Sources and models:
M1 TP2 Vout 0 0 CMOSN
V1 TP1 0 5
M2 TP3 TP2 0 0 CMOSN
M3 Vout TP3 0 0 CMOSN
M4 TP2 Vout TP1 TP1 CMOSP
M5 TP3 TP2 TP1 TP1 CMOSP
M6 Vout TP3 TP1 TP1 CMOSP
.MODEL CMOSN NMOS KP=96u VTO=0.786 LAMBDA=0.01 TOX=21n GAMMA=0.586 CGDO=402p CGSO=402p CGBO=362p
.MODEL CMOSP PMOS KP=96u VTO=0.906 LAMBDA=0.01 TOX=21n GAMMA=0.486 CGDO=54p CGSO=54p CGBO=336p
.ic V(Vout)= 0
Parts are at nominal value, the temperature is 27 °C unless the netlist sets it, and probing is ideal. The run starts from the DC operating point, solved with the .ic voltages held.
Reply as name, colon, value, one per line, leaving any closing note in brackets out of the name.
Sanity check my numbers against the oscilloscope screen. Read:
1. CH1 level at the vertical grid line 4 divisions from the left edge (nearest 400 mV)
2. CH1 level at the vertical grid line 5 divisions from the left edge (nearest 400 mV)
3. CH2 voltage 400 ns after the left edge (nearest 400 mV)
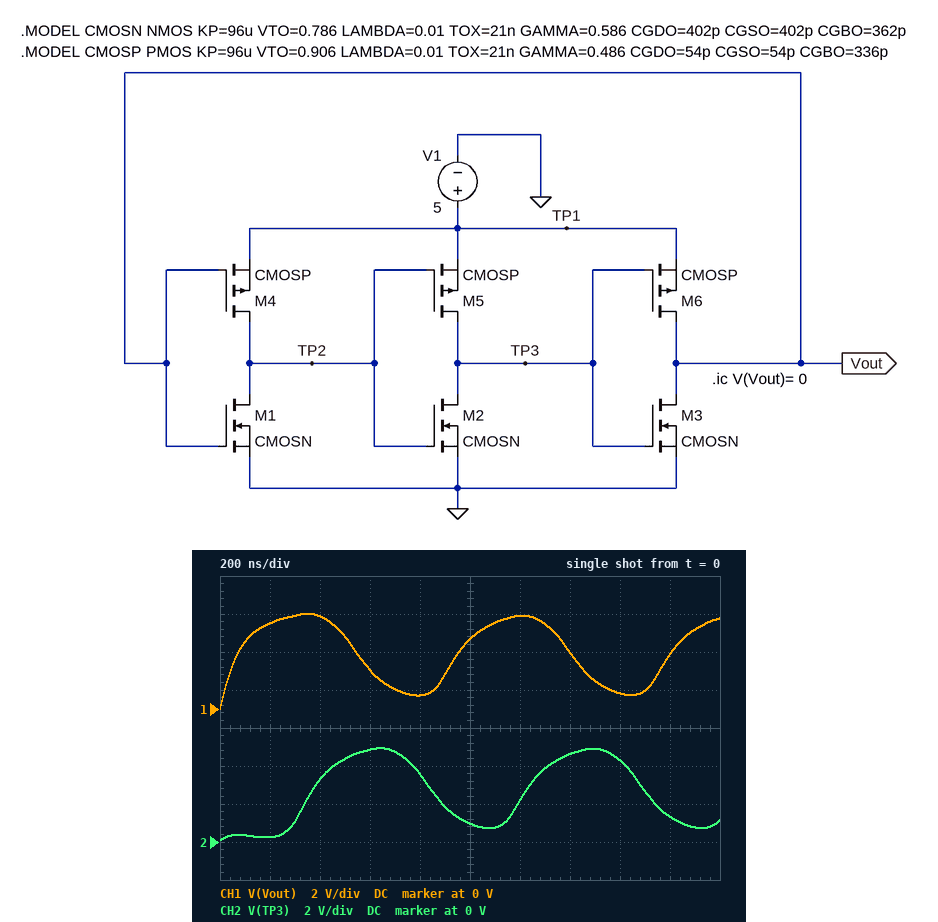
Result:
CH1 level at the vertical grid line 4 divisions from the left edge: 800 mV
CH1 level at the vertical grid line 5 divisions from the left edge: 3.6 V
CH2 voltage 400 ns after the left edge: 3.2 V
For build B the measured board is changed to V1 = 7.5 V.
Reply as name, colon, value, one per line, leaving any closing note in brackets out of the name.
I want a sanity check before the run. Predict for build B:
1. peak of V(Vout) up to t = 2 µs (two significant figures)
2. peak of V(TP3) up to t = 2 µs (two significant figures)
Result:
peak of V(Vout) up to t = 2 µs: 7.4 V
peak of V(TP3) up to t = 2 µs: 7.3 V
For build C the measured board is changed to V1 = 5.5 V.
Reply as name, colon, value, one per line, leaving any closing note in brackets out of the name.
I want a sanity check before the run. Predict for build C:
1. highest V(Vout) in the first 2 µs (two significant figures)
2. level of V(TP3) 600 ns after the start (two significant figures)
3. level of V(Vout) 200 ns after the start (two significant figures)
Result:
highest V(Vout) in the first 2 µs: 5.5 V
level of V(TP3) 600 ns after the start: 5.4 V
level of V(Vout) 200 ns after the start: 5.1 V
